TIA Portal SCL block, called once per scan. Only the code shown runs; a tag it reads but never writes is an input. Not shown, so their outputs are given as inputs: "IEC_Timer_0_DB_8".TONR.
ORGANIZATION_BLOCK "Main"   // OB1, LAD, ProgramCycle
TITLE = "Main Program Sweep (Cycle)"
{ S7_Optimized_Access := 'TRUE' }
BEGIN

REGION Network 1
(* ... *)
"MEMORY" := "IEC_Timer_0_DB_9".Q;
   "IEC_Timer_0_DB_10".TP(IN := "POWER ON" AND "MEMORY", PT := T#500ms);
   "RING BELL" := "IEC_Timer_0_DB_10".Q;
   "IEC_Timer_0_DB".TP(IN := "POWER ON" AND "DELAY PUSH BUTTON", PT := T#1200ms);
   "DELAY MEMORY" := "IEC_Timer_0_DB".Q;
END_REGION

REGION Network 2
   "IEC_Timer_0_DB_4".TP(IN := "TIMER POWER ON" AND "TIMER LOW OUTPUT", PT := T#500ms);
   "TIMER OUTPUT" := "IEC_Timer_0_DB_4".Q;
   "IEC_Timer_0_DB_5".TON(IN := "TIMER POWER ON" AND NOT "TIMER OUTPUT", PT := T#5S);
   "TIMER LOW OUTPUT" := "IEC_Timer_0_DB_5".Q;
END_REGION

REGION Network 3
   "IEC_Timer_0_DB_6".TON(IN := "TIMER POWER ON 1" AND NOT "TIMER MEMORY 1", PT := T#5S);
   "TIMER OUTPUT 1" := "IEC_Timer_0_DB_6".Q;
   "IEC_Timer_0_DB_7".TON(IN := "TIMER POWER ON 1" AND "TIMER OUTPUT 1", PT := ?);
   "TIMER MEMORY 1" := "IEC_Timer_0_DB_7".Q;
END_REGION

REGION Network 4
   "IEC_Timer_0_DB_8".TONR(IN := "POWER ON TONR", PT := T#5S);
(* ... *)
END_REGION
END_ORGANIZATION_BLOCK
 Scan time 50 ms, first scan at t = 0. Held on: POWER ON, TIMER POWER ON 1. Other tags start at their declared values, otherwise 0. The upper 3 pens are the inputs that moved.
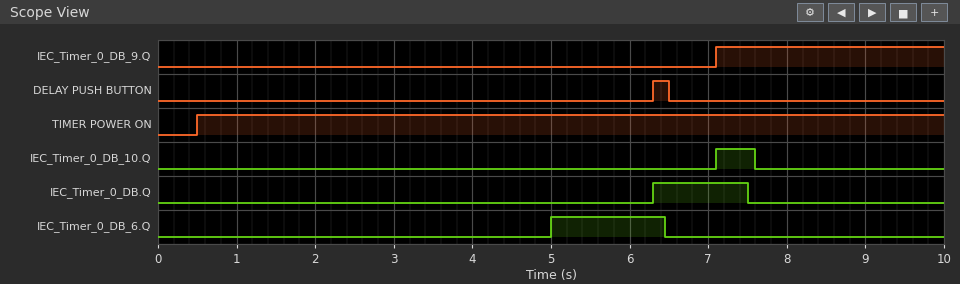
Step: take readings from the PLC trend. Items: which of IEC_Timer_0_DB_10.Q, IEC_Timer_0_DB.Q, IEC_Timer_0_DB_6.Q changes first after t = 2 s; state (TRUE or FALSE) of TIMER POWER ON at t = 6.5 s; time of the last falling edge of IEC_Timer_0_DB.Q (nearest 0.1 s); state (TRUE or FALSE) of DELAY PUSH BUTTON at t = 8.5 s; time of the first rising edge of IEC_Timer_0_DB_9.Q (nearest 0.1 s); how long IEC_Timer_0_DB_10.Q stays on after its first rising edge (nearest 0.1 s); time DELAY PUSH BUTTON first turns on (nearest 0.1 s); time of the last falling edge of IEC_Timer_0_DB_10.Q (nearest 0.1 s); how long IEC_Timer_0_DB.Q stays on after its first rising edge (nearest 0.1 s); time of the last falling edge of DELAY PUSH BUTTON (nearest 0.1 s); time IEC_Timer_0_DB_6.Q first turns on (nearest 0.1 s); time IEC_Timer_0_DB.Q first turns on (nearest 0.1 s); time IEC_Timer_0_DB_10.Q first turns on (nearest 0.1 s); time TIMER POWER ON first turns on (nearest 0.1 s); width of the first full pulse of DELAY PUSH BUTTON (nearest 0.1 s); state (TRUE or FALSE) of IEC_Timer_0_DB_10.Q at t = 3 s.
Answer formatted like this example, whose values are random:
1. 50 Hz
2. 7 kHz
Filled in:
1. IEC_Timer_0_DB_6.Q
2. TRUE
3. 7.5 s
4. FALSE
5. 7.1 s
6. 0.5 s
7. 6.3 s
8. 7.6 s
9. 1.2 s
10. 6.5 s
11. 5.0 s
12. 6.3 s
13. 7.1 s
14. 0.5 s
15. 0.2 s
16. FALSE
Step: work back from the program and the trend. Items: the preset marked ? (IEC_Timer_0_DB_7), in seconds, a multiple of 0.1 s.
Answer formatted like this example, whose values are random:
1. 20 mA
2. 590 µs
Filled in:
1. 1.4 s
